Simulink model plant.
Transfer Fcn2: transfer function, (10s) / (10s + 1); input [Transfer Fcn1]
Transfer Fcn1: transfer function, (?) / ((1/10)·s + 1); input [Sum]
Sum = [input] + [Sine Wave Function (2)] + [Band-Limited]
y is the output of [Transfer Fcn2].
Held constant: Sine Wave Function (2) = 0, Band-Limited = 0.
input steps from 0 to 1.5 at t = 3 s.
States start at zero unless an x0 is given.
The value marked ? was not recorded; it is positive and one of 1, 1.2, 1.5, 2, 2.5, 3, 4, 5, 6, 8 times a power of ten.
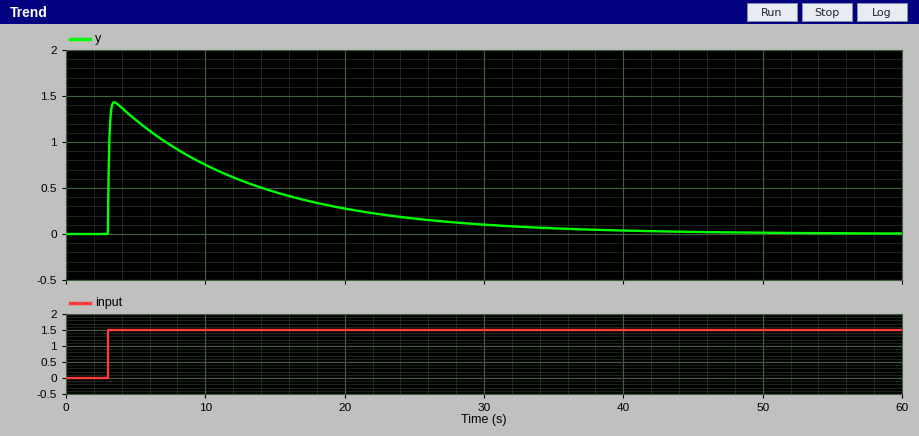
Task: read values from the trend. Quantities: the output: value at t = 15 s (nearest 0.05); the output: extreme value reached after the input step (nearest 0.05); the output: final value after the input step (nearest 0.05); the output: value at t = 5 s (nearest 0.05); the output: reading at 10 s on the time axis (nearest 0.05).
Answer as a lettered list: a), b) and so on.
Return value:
a) 0.45
b) 1.45
c) 0.00
d) 1.25
e) 0.75
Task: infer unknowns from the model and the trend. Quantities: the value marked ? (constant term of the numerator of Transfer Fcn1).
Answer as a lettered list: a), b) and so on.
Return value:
a) 1
